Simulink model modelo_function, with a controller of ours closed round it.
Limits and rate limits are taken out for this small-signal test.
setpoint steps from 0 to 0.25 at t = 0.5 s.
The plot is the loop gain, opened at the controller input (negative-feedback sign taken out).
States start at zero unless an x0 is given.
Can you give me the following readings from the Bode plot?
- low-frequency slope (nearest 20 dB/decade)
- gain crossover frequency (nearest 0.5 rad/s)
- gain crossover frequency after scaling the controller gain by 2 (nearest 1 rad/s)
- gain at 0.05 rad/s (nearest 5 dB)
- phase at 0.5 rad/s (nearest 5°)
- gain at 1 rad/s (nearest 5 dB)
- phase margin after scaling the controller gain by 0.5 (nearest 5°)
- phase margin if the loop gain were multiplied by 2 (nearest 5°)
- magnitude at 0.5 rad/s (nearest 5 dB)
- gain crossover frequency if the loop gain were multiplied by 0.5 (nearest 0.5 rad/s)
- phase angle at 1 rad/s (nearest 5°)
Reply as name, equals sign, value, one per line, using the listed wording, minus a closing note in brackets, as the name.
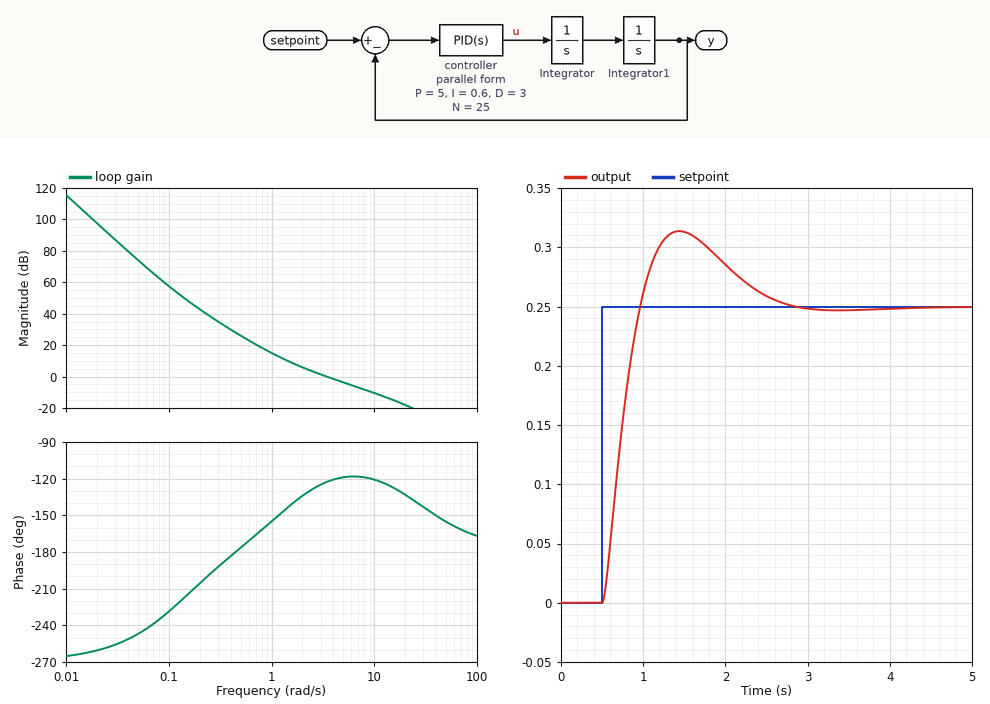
low-frequency slope = -60 dB/decade
gain crossover frequency = 3.5 rad/s
gain crossover frequency after scaling the controller gain by 2 = 6 rad/s
gain at 0.05 rad/s = 75 dB
phase at 0.5 rad/s = -175°
gain at 1 rad/s = 15 dB
phase margin after scaling the controller gain by 0.5 = 45°
phase margin if the loop gain were multiplied by 2 = 60°
magnitude at 0.5 rad/s = 25 dB
gain crossover frequency if the loop gain were multiplied by 0.5 = 2.0 rad/s
phase angle at 1 rad/s = -155°
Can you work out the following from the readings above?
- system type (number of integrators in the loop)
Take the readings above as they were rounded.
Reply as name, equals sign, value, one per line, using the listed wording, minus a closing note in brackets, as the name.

system type = 3
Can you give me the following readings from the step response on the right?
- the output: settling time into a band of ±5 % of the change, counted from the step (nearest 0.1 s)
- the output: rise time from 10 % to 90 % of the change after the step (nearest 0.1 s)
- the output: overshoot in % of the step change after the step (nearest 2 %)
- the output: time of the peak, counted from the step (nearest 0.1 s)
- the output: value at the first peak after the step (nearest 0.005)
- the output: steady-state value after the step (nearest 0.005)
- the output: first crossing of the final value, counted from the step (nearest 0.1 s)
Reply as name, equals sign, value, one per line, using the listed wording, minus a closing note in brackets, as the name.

the output: settling time into a band of ±5 % of the change, counted from the step = 1.9 s
the output: rise time from 10 % to 90 % of the change after the step = 0.3 s
the output: overshoot in % of the step change after the step = 26 %
the output: time of the peak, counted from the step = 0.9 s
the output: value at the first peak after the step = 0.315
the output: steady-state value after the step = 0.250
the output: first crossing of the final value, counted from the step = 0.5 s
